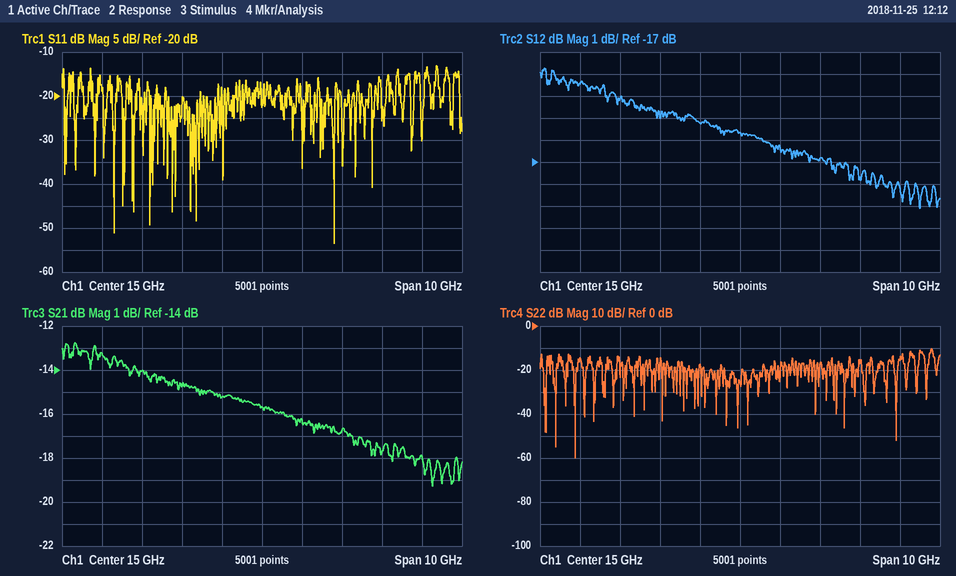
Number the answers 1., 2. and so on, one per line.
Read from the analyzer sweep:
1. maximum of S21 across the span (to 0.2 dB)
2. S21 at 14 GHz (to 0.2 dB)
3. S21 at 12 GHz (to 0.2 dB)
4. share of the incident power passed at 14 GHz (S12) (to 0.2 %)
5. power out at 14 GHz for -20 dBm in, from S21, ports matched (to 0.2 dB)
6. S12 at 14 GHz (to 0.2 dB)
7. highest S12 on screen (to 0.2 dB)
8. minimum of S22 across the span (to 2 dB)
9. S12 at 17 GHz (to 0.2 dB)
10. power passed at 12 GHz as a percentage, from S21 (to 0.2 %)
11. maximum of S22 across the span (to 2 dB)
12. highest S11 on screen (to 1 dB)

1. -12.8 dB
2. -15.2 dB
3. -14.0 dB
4. 3.0 %
5. -35.2 dBm
6. -15.2 dB
7. -12.8 dB
8. -60 dB
9. -16.8 dB
10. 4.0 %
11. -10 dB
12. -13 dB
